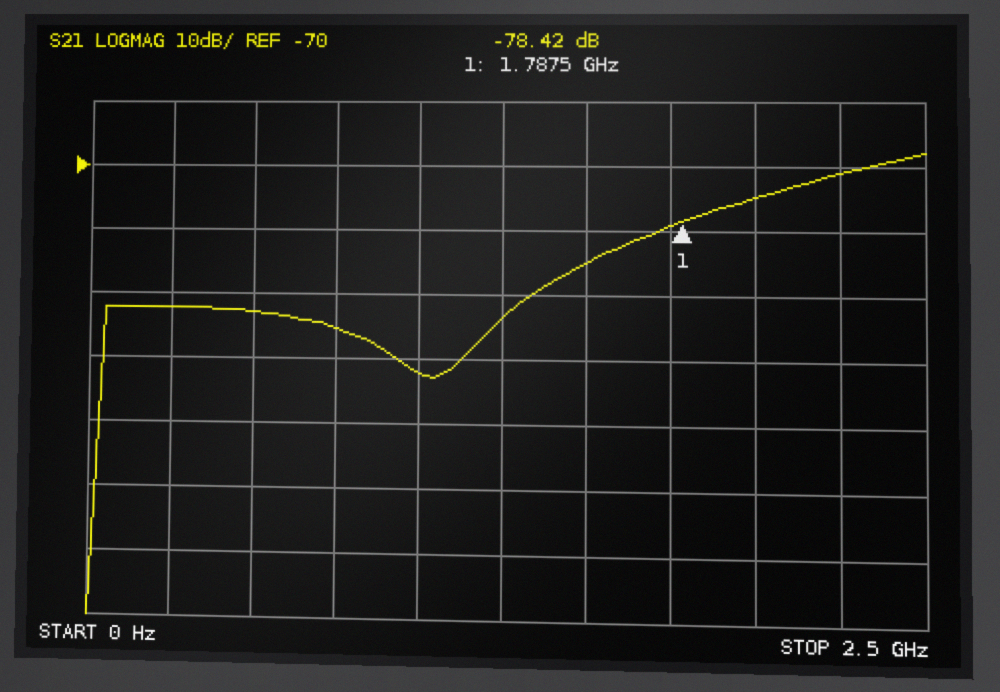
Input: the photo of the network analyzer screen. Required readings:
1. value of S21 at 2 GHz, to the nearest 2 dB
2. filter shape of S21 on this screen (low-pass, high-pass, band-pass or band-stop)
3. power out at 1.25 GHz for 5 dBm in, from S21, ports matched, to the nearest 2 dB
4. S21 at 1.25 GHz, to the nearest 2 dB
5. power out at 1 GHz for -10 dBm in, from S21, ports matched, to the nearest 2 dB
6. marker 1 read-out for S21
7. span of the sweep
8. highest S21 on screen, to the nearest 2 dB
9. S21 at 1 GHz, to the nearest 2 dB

-74 dB
high-pass
-88 dBm
-94 dB
-112 dBm
-78.42 dB
2.5 GHz
-68 dB
-102 dB
